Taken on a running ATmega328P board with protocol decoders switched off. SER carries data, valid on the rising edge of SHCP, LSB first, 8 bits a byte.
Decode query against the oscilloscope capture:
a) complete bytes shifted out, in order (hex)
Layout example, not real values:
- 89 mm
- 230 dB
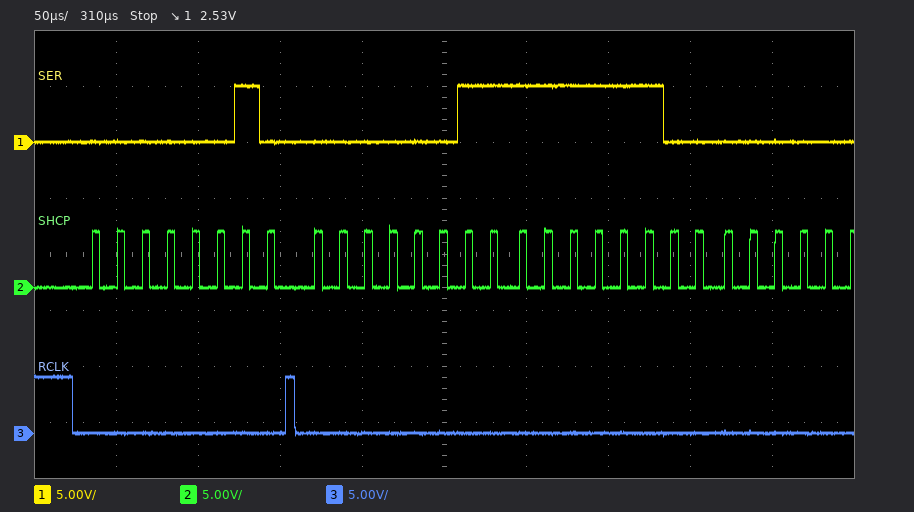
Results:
- 40 C0 3F
